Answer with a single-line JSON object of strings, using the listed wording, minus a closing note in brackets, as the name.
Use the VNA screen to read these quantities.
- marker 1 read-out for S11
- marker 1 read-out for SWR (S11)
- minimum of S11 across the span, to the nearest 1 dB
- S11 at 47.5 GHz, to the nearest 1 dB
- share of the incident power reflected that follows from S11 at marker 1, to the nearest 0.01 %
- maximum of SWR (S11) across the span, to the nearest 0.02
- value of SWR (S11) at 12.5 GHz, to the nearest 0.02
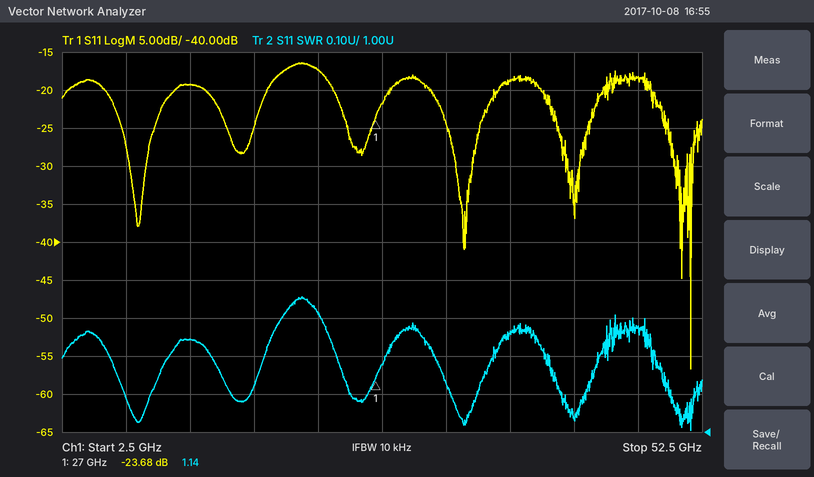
{"marker 1 read-out for S11": "-23.68 dB", "marker 1 read-out for SWR": "1.14", "minimum of S11 across the span, to the nearest 1 dB": "-57 dB", "S11 at 47.5 GHz, to the nearest 1 dB": "-18 dB", "share of the incident power reflected that follows from S11 at marker 1, to the nearest 0.01 %": "0.43 %", "maximum of SWR (S11) across the span, to the nearest 0.02": "1.36", "value of SWR (S11) at 12.5 GHz, to the nearest 0.02": "1.24"}
